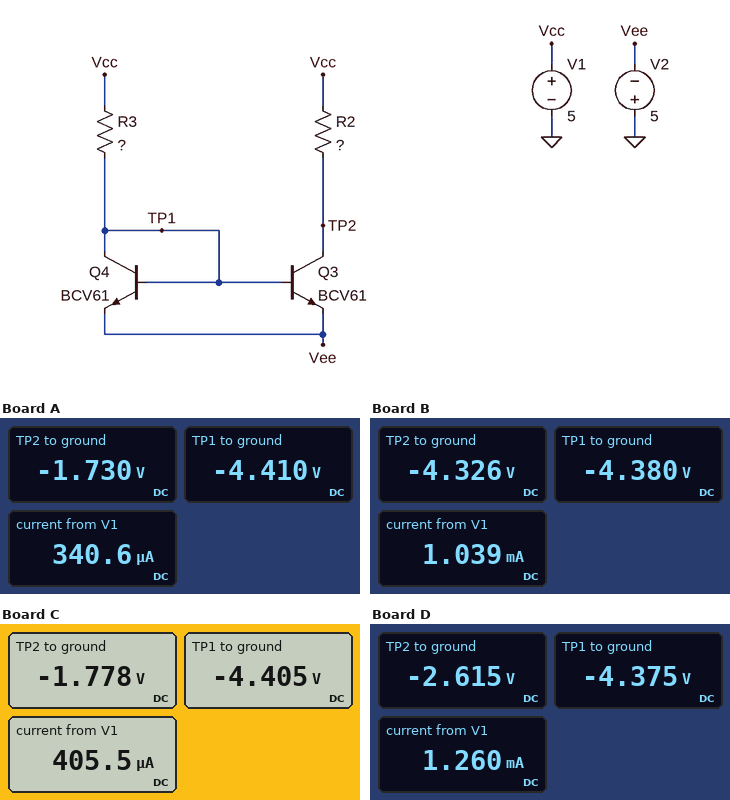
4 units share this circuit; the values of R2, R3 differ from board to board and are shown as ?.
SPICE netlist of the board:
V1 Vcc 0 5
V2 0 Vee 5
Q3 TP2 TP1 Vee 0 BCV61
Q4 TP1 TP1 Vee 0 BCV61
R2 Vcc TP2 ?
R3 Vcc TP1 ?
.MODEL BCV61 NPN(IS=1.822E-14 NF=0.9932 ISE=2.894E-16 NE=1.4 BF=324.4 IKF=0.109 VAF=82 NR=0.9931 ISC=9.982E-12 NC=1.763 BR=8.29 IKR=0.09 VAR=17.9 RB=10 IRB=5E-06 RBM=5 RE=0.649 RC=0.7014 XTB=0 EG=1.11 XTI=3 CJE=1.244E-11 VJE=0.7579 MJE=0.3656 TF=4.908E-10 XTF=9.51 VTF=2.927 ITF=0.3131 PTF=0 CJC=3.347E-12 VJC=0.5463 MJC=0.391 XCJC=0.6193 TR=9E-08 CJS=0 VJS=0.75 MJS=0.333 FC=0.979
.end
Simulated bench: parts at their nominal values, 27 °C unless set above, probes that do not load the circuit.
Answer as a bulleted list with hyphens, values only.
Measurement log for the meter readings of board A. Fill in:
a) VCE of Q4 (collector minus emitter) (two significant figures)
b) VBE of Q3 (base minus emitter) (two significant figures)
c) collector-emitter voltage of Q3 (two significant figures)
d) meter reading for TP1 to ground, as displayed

- 590 mV
- 590 mV
- 3.3 V
- -4.410 V
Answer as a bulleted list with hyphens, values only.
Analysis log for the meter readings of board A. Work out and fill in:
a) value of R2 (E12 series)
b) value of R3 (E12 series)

- 39 kΩ
- 56 kΩ
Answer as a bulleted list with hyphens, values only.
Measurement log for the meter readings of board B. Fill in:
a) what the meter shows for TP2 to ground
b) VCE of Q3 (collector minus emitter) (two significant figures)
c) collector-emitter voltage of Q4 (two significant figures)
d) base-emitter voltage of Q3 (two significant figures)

- -4.326 V
- 670 mV
- 620 mV
- 620 mV
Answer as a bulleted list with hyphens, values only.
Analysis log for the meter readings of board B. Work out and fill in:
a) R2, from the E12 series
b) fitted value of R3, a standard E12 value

- 18 kΩ
- 18 kΩ
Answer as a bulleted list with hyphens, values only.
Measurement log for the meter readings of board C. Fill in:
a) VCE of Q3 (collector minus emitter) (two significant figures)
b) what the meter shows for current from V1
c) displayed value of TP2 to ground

- 3.2 V
- 405.5 µA
- -1.778 V
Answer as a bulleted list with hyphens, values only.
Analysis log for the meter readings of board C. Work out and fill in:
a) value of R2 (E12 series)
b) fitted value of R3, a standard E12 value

- 33 kΩ
- 47 kΩ
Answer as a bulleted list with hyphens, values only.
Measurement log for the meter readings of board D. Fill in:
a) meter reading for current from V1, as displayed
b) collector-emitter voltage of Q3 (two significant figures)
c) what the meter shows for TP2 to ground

- 1.260 mA
- 2.4 V
- -2.615 V
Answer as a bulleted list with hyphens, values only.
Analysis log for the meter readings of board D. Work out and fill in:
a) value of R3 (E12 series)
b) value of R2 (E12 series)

- 15 kΩ
- 12 kΩ
